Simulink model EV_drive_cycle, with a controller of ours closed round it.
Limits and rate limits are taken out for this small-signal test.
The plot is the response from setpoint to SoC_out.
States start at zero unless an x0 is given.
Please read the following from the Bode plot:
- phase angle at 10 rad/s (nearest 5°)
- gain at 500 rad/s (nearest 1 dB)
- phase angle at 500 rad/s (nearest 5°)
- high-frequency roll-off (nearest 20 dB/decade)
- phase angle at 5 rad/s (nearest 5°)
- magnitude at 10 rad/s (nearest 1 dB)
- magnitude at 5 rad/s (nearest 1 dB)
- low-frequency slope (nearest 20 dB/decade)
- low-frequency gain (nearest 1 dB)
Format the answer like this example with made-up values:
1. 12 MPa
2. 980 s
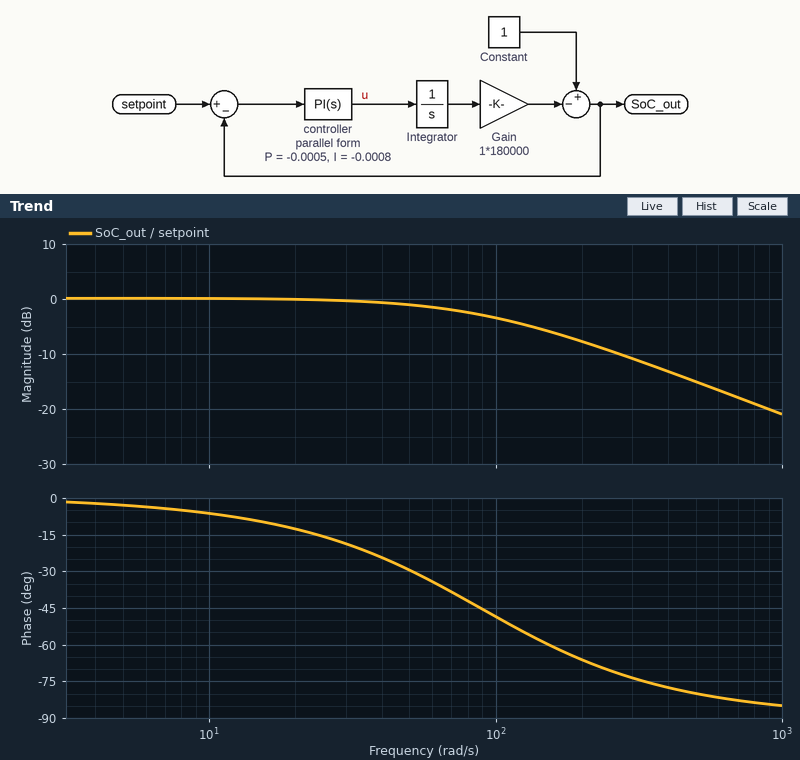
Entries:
1. -5°
2. -15 dB
3. -80°
4. -20 dB/decade
5. -5°
6. 0 dB
7. 0 dB
8. 0 dB/decade
9. 0 dB
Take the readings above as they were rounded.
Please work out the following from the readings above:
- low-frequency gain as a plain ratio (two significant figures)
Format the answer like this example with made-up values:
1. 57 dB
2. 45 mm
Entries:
1. 1.0
